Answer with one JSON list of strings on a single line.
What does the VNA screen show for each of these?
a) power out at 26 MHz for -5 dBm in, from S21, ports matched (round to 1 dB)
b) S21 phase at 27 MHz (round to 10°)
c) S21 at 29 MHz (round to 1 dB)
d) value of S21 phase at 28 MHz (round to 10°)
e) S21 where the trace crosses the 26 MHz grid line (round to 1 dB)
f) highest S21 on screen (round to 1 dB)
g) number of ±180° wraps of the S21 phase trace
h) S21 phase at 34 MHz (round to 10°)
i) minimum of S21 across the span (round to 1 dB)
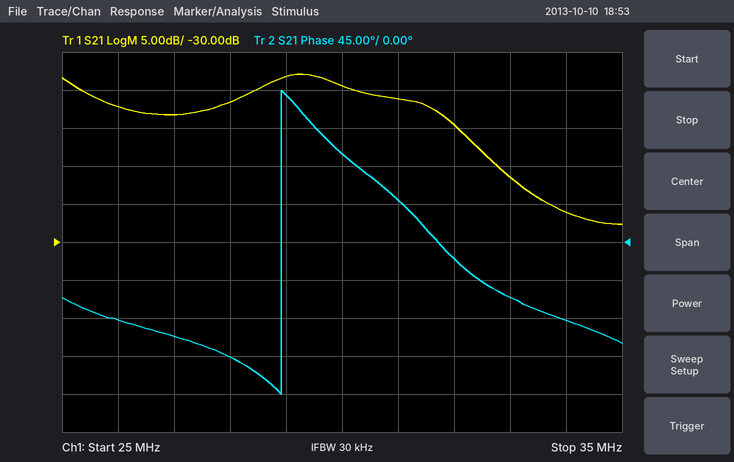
["-17 dBm", "-110°", "-8 dB", "-140°", "-12 dB", "-8 dB", "1", "-90°", "-28 dB"]
